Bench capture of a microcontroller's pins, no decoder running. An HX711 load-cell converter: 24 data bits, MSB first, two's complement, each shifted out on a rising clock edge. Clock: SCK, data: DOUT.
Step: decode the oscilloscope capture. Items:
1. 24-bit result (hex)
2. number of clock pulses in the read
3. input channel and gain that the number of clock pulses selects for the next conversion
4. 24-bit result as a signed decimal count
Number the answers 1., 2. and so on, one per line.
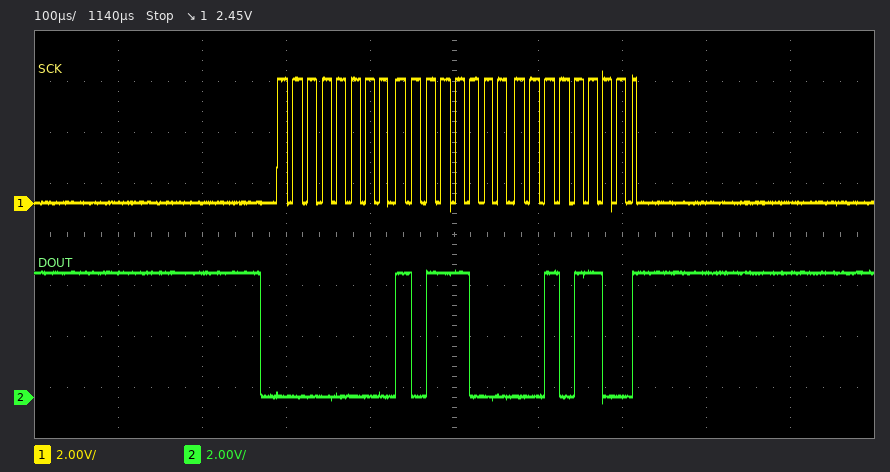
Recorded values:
1. 0x00B82C
2. 25
3. channel A, gain 128
4. 47148
